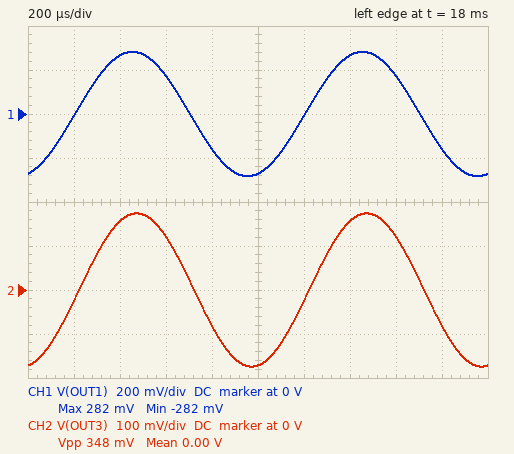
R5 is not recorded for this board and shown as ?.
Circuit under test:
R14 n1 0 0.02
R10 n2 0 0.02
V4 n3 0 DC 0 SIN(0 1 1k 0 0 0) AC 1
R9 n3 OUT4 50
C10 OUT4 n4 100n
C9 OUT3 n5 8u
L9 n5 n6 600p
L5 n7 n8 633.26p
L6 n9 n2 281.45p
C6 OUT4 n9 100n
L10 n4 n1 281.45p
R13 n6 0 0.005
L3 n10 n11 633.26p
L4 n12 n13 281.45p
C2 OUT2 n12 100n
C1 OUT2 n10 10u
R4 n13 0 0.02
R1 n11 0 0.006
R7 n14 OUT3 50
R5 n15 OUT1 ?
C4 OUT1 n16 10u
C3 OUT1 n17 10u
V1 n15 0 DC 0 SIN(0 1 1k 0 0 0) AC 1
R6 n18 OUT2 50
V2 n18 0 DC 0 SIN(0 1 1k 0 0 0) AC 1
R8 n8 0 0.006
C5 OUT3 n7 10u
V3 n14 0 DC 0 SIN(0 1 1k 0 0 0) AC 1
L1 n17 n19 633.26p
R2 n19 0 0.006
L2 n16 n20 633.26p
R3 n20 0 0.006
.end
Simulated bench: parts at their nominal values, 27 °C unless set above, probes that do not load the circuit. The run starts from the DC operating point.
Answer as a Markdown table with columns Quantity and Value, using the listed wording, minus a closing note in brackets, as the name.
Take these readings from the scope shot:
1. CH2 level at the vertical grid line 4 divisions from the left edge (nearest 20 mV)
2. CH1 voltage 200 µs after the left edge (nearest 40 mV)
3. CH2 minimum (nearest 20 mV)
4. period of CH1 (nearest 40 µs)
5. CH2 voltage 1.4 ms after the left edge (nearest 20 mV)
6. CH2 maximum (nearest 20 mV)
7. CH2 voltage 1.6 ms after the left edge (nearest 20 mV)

| Quantity | Value |
|---|---|
| CH2 level at the vertical grid line 4 divisions from the left edge | -80 mV |
| CH1 voltage 200 µs after the left edge | 0 V |
| CH2 minimum | -180 mV |
| period of CH1 | 1.00 ms |
| CH2 voltage 1.4 ms after the left edge | 160 mV |
| CH2 maximum | 180 mV |
| CH2 voltage 1.6 ms after the left edge | 120 mV |
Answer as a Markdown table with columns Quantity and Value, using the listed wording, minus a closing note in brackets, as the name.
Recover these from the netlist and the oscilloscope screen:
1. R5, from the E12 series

| Quantity | Value |
|---|---|
| R5, from the E12 series | 27 Ω |
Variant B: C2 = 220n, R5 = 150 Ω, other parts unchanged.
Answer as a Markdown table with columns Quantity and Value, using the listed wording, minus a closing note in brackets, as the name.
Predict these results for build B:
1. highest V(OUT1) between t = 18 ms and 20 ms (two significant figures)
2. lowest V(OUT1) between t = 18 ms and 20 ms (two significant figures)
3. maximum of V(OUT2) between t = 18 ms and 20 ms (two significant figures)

| Quantity | Value |
|---|---|
| highest V(OUT1) between t = 18 ms and 20 ms | 53 mV |
| lowest V(OUT1) between t = 18 ms and 20 ms | -53 mV |
| maximum of V(OUT2) between t = 18 ms and 20 ms | 300 mV |
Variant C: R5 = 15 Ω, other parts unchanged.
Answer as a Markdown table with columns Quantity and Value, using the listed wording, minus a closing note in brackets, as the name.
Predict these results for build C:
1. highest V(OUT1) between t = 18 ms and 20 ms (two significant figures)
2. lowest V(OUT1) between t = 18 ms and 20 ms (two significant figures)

| Quantity | Value |
|---|---|
| highest V(OUT1) between t = 18 ms and 20 ms | 470 mV |
| lowest V(OUT1) between t = 18 ms and 20 ms | -470 mV |
